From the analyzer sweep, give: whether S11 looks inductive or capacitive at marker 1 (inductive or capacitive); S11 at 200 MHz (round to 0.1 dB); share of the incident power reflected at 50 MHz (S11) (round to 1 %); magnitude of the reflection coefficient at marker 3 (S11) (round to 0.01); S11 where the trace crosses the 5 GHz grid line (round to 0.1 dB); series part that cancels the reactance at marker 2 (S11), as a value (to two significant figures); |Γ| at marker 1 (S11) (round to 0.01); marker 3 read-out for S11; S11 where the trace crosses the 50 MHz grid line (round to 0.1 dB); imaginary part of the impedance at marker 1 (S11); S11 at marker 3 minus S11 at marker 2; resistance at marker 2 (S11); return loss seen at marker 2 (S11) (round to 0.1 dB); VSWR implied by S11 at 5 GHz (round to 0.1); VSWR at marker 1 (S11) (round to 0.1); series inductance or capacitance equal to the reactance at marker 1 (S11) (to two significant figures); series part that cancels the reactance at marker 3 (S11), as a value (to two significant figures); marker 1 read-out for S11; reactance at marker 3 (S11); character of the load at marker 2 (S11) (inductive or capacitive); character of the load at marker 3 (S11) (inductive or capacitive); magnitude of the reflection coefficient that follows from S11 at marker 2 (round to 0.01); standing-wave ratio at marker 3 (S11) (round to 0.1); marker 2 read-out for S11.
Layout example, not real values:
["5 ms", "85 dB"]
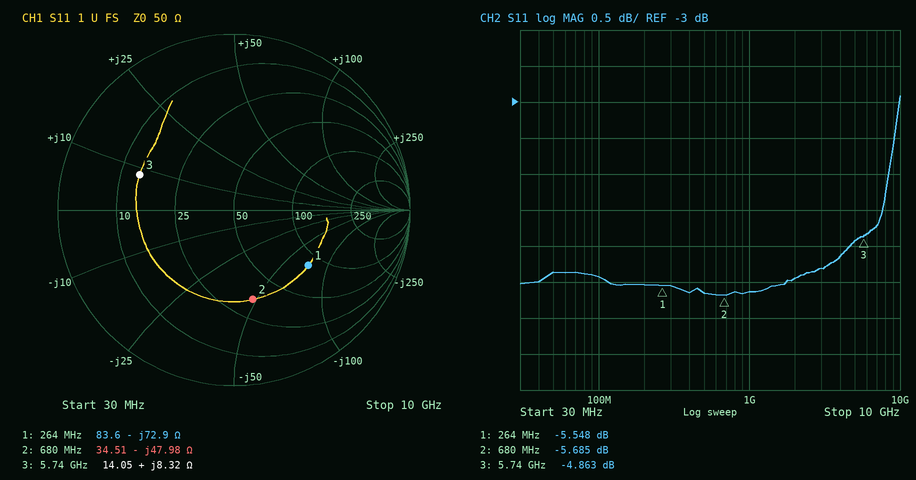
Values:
["capacitive", "-5.5 dB", "29 %", "0.57", "-4.9 dB", "11 nH", "0.53", "-4.863 dB", "-5.4 dB", "-72.9 Ω", "0.822 dB", "34.51 Ω", "5.7 dB", "3.6", "3.2", "8.3 pF", "3.3 pF", "-5.548 dB", "+8.32 Ω", "capacitive", "inductive", "0.52", "3.7", "-5.685 dB"]
